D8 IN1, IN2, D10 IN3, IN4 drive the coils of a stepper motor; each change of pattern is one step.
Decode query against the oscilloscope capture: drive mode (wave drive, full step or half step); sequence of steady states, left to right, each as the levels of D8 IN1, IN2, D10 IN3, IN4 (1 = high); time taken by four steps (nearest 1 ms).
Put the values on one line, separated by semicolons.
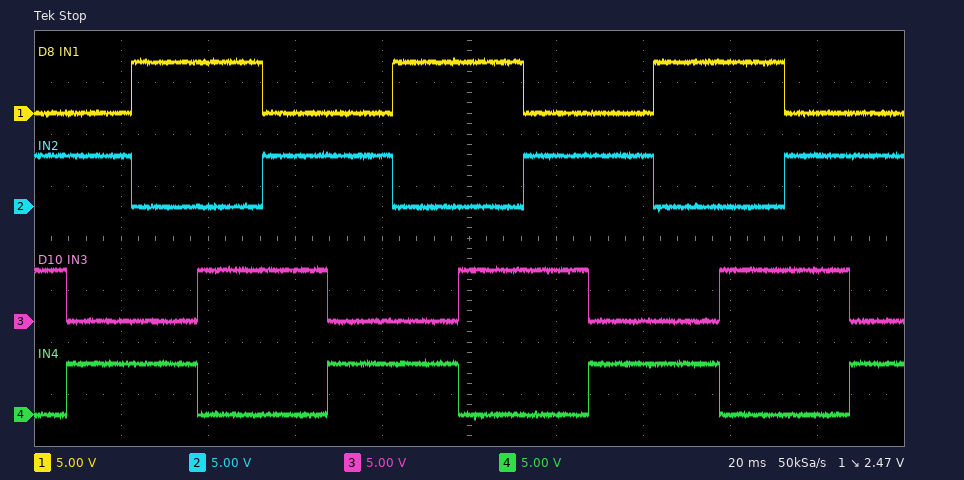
full step; 0110 0101 1001 1010 0110 0101 1001 1010 0110 0101 1001 1010 0110 0101; 60 ms
